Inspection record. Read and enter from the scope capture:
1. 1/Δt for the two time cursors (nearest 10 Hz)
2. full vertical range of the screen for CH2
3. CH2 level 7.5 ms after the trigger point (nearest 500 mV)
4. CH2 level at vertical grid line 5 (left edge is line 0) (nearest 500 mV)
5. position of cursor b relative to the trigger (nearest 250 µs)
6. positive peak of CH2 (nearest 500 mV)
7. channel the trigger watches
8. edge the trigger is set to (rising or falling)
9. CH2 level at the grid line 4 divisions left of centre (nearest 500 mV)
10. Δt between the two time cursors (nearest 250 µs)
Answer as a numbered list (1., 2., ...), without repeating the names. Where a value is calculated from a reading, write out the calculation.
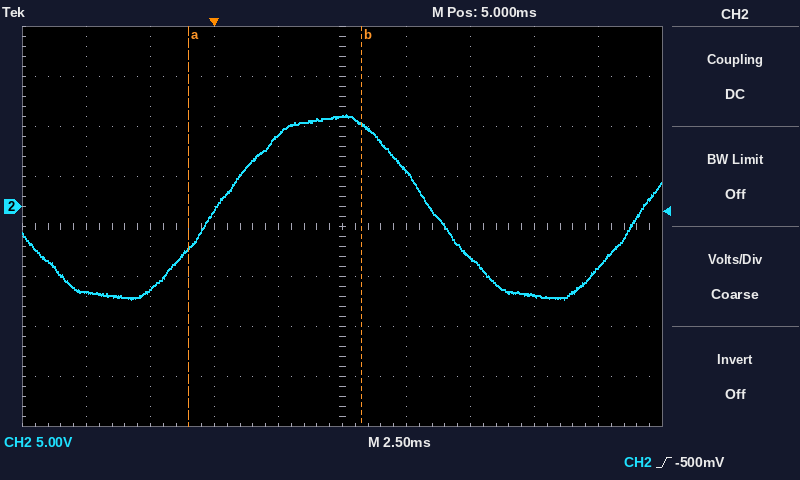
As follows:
1. 1 / 6.75 ms ≈ 150 Hz
2. 40 V
3. 3.5 V
4. 9.0 V
5. +5.75 ms
6. 9.0 V
7. CH2
8. rising
9. -8.5 V
10. 6.75 ms
